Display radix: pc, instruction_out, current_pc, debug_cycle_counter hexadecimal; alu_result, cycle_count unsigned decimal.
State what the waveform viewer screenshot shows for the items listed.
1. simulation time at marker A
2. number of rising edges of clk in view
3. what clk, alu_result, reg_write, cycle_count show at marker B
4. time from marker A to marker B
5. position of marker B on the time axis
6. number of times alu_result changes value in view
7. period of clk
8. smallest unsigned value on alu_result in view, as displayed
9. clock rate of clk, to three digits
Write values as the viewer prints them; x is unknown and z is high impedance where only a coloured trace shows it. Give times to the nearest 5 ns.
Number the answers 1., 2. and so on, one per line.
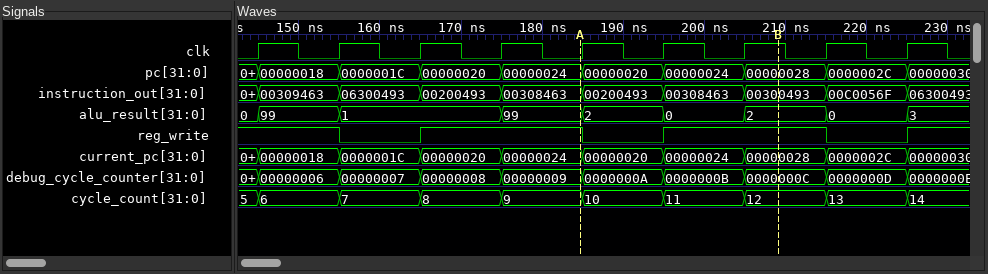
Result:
1. 185 ns
2. 9
3. clk=1, alu_result=2, reg_write=1, cycle_count=12
4. 25 ns
5. 210 ns
6. 8
7. 10 ns
8. 0
9. 100 MHz
